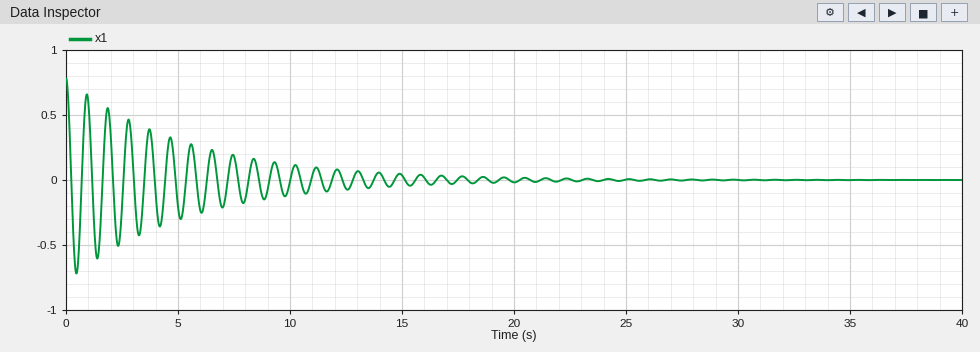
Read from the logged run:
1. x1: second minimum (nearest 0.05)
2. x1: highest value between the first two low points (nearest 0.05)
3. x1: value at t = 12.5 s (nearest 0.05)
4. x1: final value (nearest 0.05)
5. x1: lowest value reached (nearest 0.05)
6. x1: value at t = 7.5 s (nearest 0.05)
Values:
-0.60
0.65
-0.05
0.00
-0.70
0.20
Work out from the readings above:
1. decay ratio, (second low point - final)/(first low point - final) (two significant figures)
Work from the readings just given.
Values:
0.86
